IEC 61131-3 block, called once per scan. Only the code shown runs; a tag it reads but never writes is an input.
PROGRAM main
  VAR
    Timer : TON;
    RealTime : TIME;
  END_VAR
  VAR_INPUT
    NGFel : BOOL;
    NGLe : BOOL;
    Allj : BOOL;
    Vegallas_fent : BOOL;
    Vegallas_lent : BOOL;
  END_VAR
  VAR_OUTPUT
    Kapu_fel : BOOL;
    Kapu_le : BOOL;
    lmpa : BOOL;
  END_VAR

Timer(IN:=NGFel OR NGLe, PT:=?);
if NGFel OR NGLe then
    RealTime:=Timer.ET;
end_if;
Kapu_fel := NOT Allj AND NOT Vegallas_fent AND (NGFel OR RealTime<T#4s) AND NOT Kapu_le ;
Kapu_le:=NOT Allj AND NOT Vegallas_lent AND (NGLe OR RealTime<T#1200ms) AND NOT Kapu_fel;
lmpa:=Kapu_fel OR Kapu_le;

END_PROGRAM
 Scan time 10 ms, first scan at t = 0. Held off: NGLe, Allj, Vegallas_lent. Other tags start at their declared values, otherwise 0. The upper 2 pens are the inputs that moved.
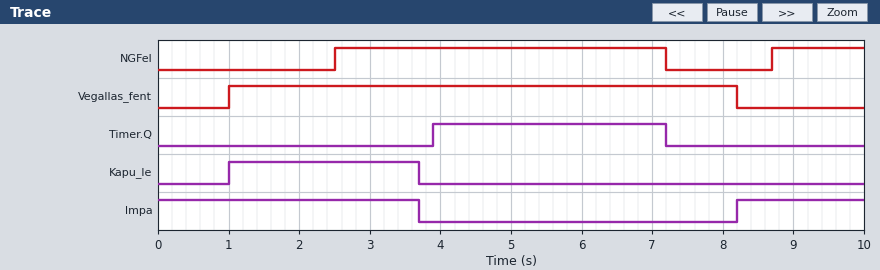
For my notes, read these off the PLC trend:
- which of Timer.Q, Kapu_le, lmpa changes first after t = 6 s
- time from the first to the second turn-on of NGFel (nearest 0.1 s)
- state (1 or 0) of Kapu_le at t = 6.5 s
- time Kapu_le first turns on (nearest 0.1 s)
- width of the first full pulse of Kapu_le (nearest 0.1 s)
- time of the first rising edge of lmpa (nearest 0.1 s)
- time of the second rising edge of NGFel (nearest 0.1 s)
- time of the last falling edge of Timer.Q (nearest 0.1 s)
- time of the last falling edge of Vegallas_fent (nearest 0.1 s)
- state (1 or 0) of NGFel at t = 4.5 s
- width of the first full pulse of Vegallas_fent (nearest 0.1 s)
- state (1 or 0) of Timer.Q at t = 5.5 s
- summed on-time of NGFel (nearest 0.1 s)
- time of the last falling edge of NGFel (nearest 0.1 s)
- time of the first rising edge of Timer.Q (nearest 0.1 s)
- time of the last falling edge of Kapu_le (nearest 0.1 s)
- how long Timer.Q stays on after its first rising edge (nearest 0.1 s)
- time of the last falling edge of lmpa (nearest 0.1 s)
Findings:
Timer.Q
6.2 s
0
1.0 s
2.7 s
8.2 s
8.7 s
7.2 s
8.2 s
1
7.2 s
1
6.0 s
7.2 s
3.9 s
3.7 s
3.3 s
3.7 s
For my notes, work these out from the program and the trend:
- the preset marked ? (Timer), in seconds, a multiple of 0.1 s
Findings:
1.4 s
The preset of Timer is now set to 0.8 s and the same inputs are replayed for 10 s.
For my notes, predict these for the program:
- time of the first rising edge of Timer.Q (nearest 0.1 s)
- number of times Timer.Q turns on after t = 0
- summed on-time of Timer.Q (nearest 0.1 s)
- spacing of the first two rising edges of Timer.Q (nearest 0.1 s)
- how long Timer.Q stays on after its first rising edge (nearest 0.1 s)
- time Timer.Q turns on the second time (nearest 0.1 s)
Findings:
3.3 s
2
4.4 s
6.2 s
3.9 s
9.5 s
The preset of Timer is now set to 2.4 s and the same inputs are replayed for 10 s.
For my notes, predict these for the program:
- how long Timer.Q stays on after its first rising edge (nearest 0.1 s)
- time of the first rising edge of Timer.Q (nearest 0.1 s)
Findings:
2.3 s
4.9 s
